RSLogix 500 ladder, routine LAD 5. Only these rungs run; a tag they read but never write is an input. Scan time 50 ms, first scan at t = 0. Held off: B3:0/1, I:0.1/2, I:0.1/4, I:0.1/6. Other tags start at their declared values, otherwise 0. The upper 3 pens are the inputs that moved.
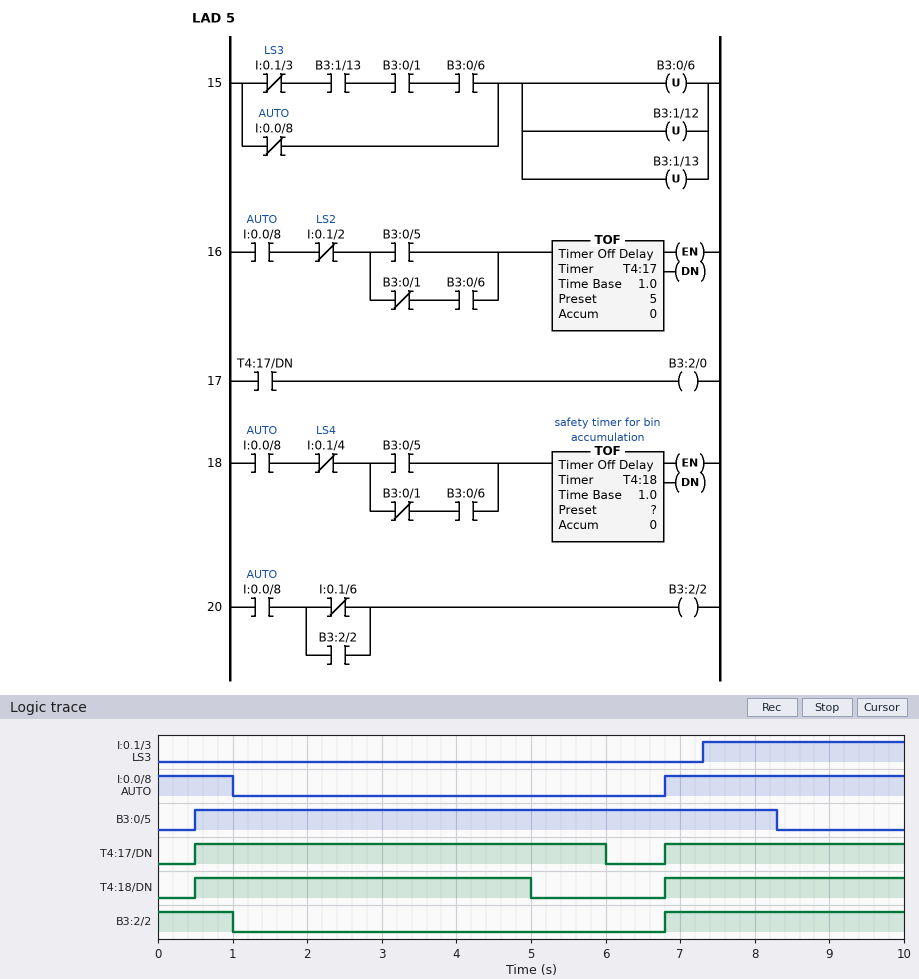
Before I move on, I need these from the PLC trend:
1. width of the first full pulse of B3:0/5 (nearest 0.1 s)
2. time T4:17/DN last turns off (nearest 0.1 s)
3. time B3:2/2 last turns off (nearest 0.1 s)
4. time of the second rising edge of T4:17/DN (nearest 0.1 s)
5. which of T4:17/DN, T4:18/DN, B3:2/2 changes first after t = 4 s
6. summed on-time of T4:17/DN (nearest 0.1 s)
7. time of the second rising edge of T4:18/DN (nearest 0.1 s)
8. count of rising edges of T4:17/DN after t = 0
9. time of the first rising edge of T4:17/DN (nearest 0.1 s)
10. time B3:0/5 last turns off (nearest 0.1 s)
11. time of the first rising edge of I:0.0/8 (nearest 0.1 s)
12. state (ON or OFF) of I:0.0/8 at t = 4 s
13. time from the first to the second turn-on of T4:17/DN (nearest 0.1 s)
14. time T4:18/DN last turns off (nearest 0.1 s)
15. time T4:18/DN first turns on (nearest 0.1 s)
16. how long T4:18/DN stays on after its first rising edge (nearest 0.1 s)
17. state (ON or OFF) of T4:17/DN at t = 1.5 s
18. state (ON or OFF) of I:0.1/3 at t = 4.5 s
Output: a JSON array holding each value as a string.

["7.8 s", "6.0 s", "1.0 s", "6.8 s", "T4:18/DN", "8.7 s", "6.8 s", "2", "0.5 s", "8.3 s", "6.8 s", "OFF", "6.3 s", "5.0 s", "0.5 s", "4.5 s", "ON", "OFF"]
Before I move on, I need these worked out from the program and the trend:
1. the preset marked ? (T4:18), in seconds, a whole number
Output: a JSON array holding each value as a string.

["4 s"]
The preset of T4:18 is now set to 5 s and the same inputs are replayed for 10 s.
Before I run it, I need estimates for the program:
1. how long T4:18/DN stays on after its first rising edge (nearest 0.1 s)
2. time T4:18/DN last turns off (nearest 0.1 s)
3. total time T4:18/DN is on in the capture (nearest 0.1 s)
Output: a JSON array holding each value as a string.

["5.5 s", "6.0 s", "8.7 s"]
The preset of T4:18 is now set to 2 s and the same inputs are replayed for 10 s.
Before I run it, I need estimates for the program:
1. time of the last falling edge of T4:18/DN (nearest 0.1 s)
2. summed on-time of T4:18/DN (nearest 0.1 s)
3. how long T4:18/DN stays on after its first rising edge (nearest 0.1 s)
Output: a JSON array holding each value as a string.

["3.0 s", "5.7 s", "2.5 s"]
